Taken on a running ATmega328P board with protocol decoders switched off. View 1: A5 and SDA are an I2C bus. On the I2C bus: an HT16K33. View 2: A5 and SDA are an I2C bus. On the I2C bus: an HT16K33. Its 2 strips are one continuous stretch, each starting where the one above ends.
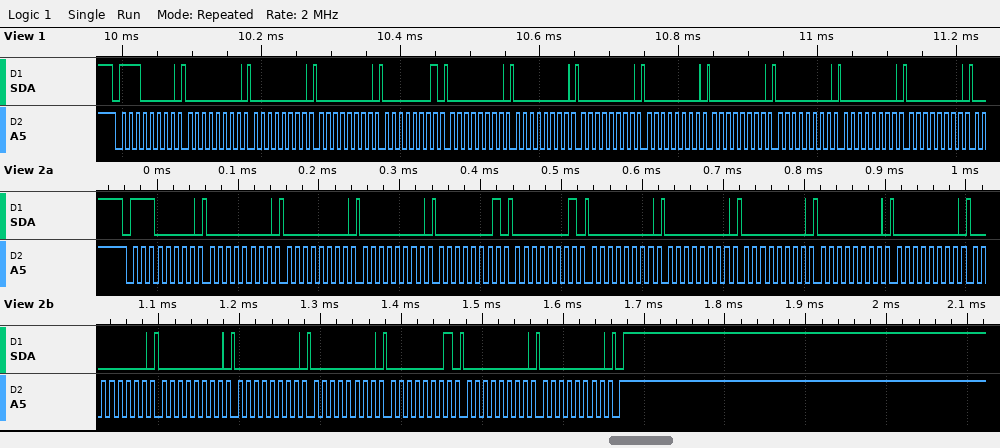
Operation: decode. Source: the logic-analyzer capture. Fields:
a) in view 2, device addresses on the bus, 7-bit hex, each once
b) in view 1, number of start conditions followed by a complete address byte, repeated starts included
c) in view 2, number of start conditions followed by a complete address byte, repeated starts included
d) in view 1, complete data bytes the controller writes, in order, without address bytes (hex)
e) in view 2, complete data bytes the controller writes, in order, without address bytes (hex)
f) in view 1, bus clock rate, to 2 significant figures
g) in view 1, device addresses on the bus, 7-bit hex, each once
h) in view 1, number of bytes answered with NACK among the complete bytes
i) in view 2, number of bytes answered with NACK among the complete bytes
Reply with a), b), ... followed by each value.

a) 0x70
b) 1
c) 1
d) 00 00 00 01 00 00 00 00 00 00 00 00
e) 00 00 00 01 01 00 00 00 00 00 00 00 00 00 01 00 00
f) 100 kHz
g) 0x70
h) 0
i) 0
